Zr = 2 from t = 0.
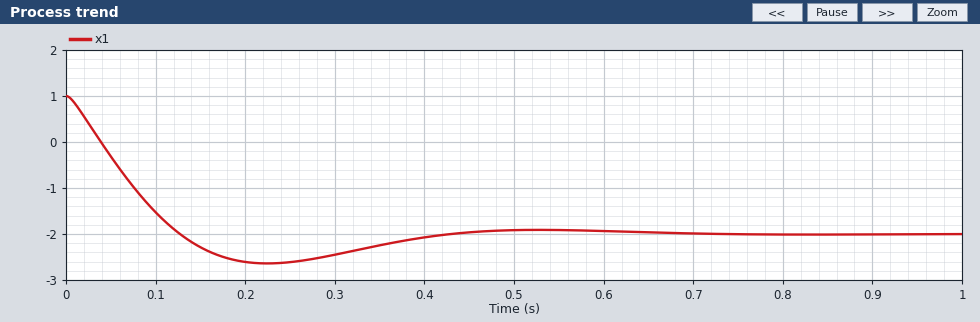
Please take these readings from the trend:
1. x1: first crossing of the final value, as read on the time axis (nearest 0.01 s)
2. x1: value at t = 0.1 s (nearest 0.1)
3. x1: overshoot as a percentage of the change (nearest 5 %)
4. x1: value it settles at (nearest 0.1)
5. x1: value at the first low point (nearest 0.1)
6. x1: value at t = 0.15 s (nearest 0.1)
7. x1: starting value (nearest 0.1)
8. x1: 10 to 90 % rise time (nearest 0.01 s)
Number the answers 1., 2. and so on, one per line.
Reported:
1. 0.13 s
2. -1.5
3. 20 %
4. -2.0
5. -2.6
6. -2.3
7. 1.0
8. 0.09 s
